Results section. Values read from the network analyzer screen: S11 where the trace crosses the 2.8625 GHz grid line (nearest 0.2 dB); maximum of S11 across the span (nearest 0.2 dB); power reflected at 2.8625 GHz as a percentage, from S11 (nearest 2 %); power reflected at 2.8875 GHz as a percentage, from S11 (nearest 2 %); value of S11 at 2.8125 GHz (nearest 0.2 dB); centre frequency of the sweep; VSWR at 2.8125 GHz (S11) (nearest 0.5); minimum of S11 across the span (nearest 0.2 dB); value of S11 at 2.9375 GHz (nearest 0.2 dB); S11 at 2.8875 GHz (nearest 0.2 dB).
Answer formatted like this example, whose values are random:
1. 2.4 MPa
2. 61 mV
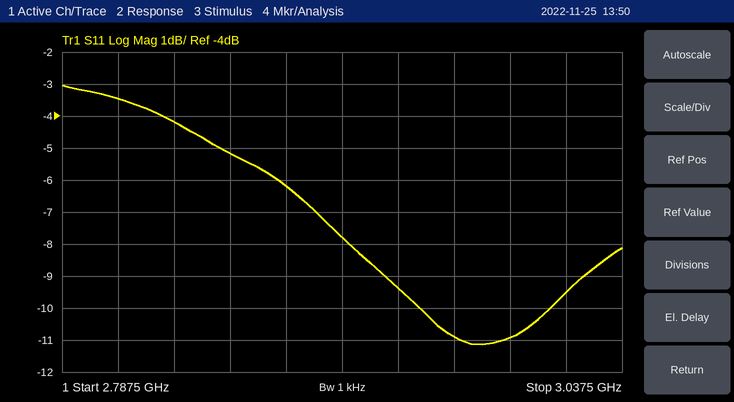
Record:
1. -5.2 dB
2. -3.0 dB
3. 30 %
4. 24 %
5. -3.4 dB
6. 2.9125 GHz
7. 5.0
8. -11.2 dB
9. -9.4 dB
10. -6.2 dB
